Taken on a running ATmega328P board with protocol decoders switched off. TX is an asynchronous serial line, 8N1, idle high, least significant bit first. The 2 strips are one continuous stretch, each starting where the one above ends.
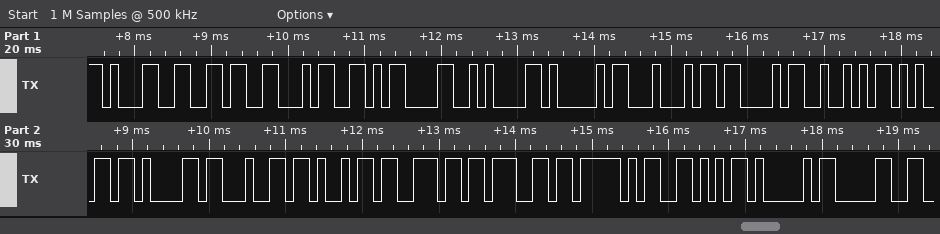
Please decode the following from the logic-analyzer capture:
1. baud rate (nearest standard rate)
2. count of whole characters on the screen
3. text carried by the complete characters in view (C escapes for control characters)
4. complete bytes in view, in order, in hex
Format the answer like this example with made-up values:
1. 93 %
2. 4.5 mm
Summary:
1. 9600 baud
2. 19
3. "164\r\nADCReading_VA0"
4. 0x31 0x36 0x34 0x0D 0x0A 0x41 0x44 0x43 0x52 0x65 0x61 0x64 0x69 0x6E 0x67 0x5F 0x56 0x41 0x30
